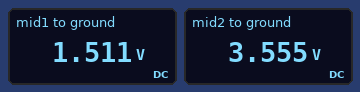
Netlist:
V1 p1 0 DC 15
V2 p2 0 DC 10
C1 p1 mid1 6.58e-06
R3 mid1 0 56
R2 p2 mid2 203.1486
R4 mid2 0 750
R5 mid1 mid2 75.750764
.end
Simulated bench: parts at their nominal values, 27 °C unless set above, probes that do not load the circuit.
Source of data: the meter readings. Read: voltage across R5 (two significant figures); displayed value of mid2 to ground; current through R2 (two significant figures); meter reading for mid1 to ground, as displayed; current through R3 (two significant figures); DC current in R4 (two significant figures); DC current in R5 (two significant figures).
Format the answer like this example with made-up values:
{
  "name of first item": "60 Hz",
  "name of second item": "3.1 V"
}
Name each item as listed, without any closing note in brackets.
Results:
{
  "voltage across R5": "2.0 V",
  "displayed value of mid2 to ground": "3.555 V",
  "current through R2": "32 mA",
  "meter reading for mid1 to ground, as displayed": "1.511 V",
  "current through R3": "27 mA",
  "DC current in R4": "4.7 mA",
  "DC current in R5": "27 mA"
}
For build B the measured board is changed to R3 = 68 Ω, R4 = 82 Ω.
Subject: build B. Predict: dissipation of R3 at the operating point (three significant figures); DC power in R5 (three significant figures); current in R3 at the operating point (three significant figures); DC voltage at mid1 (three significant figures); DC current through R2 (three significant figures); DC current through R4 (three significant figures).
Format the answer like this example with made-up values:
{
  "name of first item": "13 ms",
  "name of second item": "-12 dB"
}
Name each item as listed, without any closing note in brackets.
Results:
{
  "dissipation of R3 at the operating point": "13.8 mW",
  "DC power in R5": "15.3 mW",
  "current in R3 at the operating point": "14.2 mA",
  "DC voltage at mid1": "967 mV",
  "DC current through R2": "39.2 mA",
  "DC current through R4": "24.9 mA"
}
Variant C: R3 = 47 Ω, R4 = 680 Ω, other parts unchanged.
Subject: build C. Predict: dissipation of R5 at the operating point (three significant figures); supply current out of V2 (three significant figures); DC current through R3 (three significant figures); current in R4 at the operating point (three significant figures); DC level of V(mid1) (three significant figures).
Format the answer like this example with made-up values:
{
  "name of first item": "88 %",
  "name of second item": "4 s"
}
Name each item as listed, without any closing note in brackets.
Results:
{
  "dissipation of R5 at the operating point": "57.6 mW",
  "supply current out of V2": "32.6 mA",
  "DC current through R3": "27.6 mA",
  "current in R4 at the operating point": "4.98 mA",
  "DC level of V(mid1)": "1.30 V"
}
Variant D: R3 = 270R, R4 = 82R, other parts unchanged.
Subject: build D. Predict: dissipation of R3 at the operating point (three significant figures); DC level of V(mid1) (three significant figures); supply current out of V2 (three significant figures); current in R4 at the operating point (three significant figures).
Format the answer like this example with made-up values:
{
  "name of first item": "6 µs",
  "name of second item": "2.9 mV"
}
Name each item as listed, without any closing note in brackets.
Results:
{
  "dissipation of R3 at the operating point": "13.7 mW",
  "DC level of V(mid1)": "1.92 V",
  "supply current out of V2": "37.1 mA",
  "current in R4 at the operating point": "30.0 mA"
}
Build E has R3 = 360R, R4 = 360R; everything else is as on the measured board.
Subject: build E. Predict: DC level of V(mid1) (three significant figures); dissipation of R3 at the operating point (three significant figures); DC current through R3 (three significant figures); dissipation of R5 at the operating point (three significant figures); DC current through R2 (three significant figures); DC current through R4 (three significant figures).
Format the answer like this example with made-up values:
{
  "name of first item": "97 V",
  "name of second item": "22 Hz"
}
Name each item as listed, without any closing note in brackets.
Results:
{
  "DC level of V(mid1)": "4.07 V",
  "dissipation of R3 at the operating point": "46.0 mW",
  "DC current through R3": "11.3 mA",
  "dissipation of R5 at the operating point": "9.68 mW",
  "DC current through R2": "25.0 mA",
  "DC current through R4": "13.7 mA"
}
